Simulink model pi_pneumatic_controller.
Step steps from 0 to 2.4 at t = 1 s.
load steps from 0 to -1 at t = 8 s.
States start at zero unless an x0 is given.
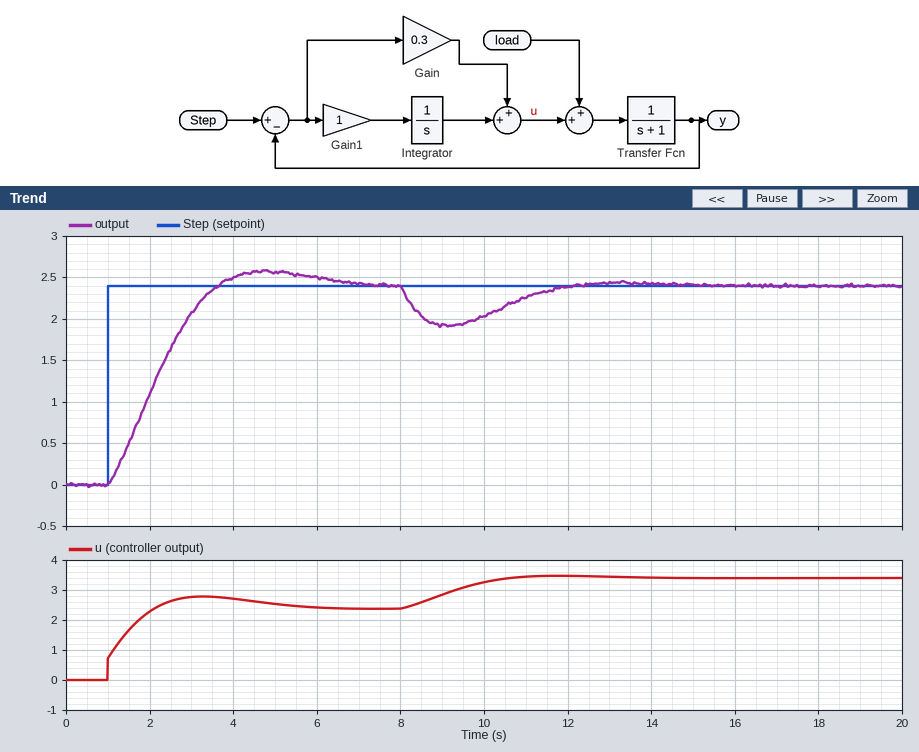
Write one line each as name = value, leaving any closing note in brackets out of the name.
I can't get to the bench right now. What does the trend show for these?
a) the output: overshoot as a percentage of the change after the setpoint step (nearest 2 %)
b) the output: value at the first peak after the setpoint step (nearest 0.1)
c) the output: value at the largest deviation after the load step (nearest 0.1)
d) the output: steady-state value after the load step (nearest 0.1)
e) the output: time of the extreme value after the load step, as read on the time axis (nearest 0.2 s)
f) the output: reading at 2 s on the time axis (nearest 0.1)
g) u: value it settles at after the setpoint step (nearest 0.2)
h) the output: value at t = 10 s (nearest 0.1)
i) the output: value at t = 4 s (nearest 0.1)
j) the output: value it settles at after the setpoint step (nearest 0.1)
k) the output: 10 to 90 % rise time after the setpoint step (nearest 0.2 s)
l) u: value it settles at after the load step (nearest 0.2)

the output: overshoot as a percentage of the change after the setpoint step = 8 %
the output: value at the first peak after the setpoint step = 2.6
the output: value at the largest deviation after the load step = 1.9
the output: steady-state value after the load step = 2.4
the output: time of the extreme value after the load step, as read on the time axis = 9.2 s
the output: reading at 2 s on the time axis = 1.1
u: value it settles at after the setpoint step = 2.4
the output: value at t = 10 s = 2.0
the output: value at t = 4 s = 2.5
the output: value it settles at after the setpoint step = 2.4
the output: 10 to 90 % rise time after the setpoint step = 1.8 s
u: value it settles at after the load step = 3.4
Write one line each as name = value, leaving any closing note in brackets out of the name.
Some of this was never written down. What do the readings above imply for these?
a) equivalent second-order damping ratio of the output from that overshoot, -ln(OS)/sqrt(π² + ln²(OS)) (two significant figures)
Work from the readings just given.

equivalent second-order damping ratio of the output from that overshoot, -ln(OS)/sqrt(π² + ln²(OS)) = 0.63
